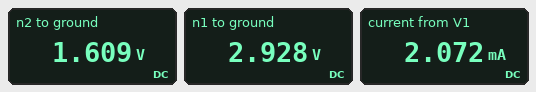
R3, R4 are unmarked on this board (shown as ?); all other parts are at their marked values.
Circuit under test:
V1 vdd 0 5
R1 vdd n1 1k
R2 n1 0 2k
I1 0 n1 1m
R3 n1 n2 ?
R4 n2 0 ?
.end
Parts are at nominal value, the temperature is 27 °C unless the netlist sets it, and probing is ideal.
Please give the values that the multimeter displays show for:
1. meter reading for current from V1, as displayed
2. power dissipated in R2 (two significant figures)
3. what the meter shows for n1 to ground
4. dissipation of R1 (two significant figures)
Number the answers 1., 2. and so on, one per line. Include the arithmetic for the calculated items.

1. 2.072 mA
2. (2.928 V)^2 / 2 kΩ = 4.3 mW
3. 2.928 V
4. (5 V - 2.928 V)^2 / 1 kΩ = 4.3 mW
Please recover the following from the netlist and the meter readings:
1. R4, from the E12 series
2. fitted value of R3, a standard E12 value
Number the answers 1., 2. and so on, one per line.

1. 1 kΩ
2. 820 Ω
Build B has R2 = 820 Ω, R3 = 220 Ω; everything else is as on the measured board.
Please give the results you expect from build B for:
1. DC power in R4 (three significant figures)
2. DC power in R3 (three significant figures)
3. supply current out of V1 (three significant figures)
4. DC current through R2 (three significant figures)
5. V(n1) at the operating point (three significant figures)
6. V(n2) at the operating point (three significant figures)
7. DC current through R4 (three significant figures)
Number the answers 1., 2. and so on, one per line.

1. 2.62 mW
2. 576 µW
3. 3.03 mA
4. 2.41 mA
5. 1.97 V
6. 1.62 V
7. 1.62 mA
